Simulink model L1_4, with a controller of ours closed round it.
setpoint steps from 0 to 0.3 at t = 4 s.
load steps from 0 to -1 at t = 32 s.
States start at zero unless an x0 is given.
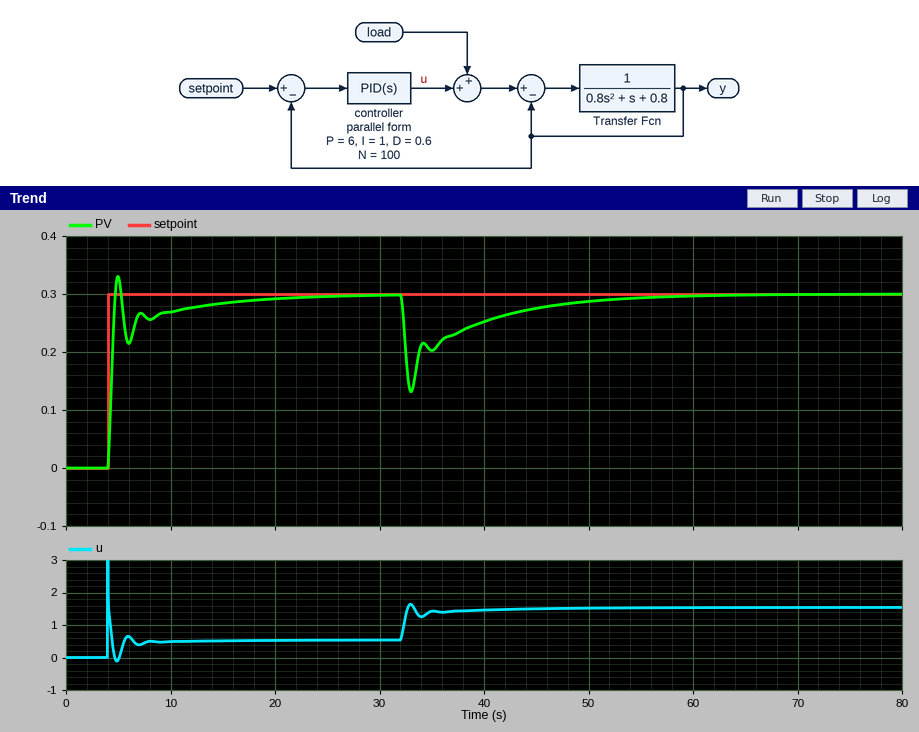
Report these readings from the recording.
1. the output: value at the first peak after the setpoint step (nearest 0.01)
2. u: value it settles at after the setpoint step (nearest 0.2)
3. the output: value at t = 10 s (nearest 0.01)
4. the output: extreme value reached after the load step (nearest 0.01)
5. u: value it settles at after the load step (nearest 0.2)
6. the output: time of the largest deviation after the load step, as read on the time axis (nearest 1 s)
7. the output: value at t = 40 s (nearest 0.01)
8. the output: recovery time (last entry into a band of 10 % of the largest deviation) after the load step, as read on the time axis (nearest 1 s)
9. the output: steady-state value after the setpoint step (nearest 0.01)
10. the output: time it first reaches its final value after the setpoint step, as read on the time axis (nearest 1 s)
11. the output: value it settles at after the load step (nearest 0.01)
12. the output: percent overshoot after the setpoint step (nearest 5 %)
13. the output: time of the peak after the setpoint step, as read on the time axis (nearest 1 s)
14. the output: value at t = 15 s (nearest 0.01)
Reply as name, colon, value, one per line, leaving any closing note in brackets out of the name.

the output: value at the first peak after the setpoint step: 0.33
u: value it settles at after the setpoint step: 0.6
the output: value at t = 10 s: 0.27
the output: extreme value reached after the load step: 0.13
u: value it settles at after the load step: 1.6
the output: time of the largest deviation after the load step, as read on the time axis: 33 s
the output: value at t = 40 s: 0.25
the output: recovery time (last entry into a band of 10 % of the largest deviation) after the load step, as read on the time axis: 48 s
the output: steady-state value after the setpoint step: 0.30
the output: time it first reaches its final value after the setpoint step, as read on the time axis: 5 s
the output: value it settles at after the load step: 0.30
the output: percent overshoot after the setpoint step: 10 %
the output: time of the peak after the setpoint step, as read on the time axis: 5 s
the output: value at t = 15 s: 0.28
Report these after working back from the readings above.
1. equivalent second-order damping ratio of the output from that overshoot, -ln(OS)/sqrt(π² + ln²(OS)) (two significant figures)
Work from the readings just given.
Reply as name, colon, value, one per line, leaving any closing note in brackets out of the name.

equivalent second-order damping ratio of the output from that overshoot, -ln(OS)/sqrt(π² + ln²(OS)): 0.59
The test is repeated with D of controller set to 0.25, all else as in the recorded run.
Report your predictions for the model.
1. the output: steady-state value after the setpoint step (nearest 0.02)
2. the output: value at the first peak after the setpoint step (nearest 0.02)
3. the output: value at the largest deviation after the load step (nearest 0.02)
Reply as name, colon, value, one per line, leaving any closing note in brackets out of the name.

the output: steady-state value after the setpoint step: 0.30
the output: value at the first peak after the setpoint step: 0.36
the output: value at the largest deviation after the load step: 0.12
